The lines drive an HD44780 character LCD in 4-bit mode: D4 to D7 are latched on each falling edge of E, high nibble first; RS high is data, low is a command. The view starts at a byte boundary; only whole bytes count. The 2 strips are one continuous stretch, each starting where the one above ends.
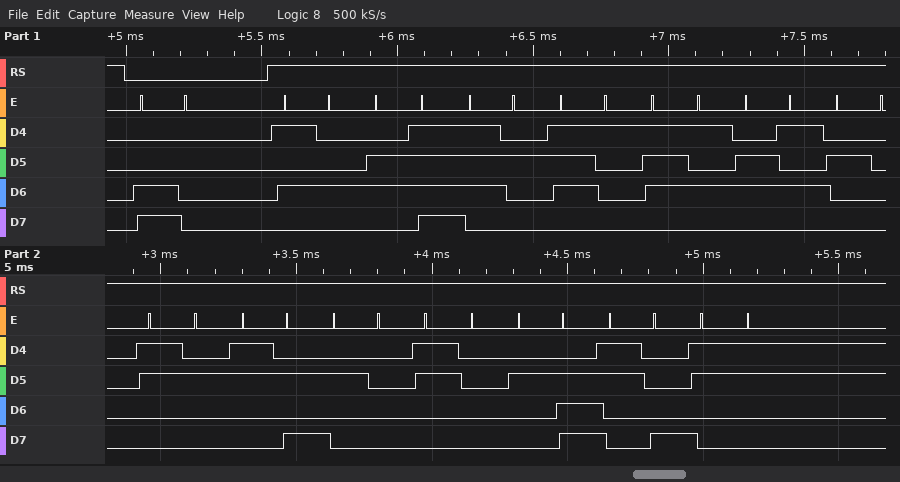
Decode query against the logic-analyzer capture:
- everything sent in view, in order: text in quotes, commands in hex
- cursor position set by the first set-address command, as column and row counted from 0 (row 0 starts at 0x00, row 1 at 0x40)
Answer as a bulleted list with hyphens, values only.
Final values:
- 0xC0 "Torque 2: 0.83"
- column 0, row 1
